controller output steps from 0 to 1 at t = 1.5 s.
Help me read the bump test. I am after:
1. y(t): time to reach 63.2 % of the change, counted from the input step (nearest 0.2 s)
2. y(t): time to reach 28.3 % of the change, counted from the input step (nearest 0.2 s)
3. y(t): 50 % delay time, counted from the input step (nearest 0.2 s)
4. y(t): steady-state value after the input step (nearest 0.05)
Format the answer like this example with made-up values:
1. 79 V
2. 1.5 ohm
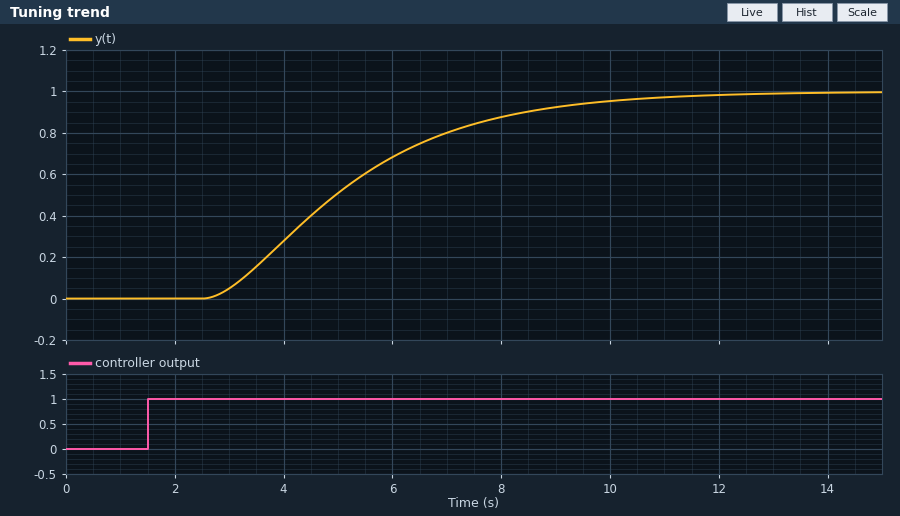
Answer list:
1. 4.2 s
2. 2.6 s
3. 3.4 s
4. 1.00
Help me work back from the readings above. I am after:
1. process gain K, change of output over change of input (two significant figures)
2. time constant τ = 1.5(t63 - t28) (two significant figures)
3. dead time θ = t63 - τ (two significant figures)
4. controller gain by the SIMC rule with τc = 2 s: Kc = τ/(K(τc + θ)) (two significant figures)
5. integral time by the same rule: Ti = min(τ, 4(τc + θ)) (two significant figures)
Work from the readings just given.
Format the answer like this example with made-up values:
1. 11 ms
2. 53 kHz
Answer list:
1. 1.0
2. 2.4 s
3. 1.8 s
4. 0.63
5. 2.4 s
